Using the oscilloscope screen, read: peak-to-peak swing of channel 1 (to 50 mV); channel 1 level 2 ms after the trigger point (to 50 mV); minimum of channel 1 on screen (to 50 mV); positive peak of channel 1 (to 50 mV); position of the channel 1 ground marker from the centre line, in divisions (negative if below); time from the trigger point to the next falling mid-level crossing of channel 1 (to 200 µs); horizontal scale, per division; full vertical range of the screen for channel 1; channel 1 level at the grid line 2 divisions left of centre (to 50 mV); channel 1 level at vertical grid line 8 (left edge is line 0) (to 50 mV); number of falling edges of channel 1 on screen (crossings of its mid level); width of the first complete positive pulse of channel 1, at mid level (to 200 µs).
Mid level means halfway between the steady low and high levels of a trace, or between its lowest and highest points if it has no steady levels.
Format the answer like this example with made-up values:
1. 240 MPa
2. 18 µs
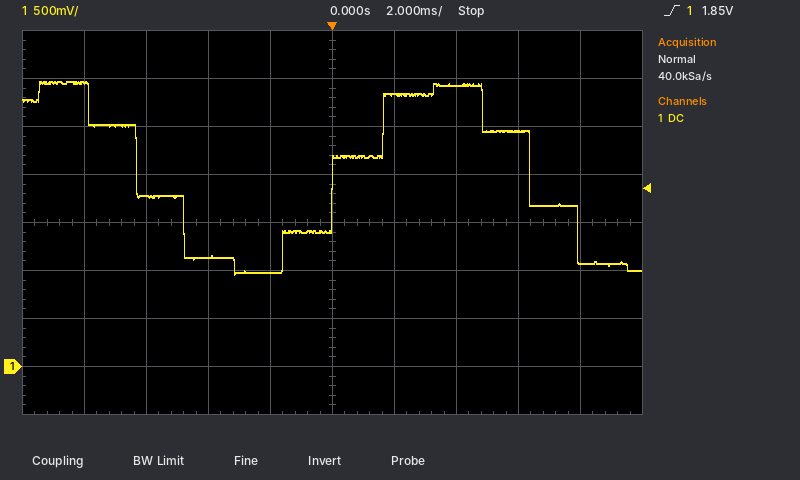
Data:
1. 2.00 V
2. 2.85 V
3. 950 mV
4. 2.95 V
5. -3.0 div
6. 6.4 ms
7. 2 ms
8. 4 V
9. 1.15 V
10. 2.45 V
11. 2
12. 6.4 ms
